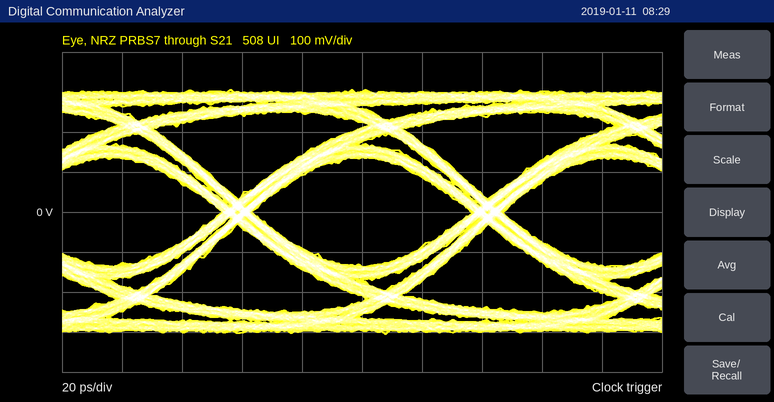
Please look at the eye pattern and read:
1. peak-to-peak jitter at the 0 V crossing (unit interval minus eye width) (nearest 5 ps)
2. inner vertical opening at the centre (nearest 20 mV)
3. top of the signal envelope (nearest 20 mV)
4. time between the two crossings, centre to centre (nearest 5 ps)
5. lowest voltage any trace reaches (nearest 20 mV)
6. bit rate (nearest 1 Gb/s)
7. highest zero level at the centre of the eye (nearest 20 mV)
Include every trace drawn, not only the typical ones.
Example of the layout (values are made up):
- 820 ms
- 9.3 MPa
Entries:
- 10 ps
- 280 mV
- 300 mV
- 85 ps
- -300 mV
- 12 Gb/s
- -140 mV
